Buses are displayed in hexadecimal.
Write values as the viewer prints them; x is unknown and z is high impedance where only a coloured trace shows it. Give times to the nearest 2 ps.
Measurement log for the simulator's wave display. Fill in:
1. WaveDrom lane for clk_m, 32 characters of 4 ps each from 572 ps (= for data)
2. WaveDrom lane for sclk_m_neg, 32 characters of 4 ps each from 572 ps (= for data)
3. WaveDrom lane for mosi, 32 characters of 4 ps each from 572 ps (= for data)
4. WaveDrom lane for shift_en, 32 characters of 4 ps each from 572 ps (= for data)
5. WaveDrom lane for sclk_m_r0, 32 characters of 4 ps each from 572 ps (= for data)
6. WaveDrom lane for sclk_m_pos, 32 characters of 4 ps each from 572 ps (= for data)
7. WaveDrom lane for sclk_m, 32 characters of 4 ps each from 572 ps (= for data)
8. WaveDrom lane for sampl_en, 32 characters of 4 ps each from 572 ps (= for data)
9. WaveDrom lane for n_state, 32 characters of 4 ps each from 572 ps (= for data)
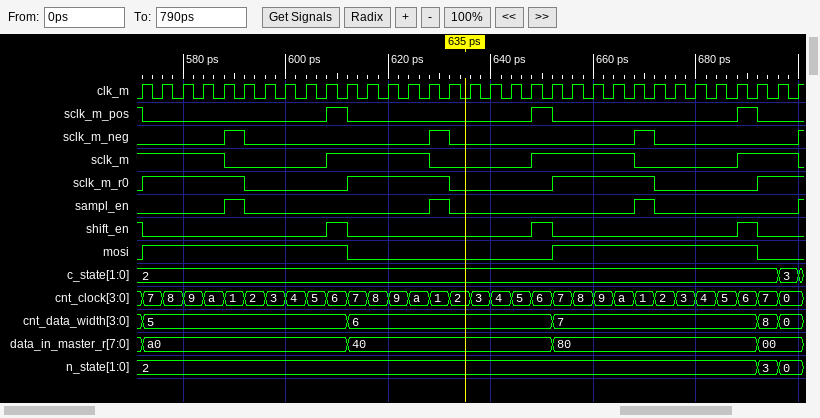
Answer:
{name: 'clk_m', wave: 'p...............................'}
{name: 'sclk_m_neg', wave: '0...10........10........10......'}
{name: 'mosi', wave: '1.........0.........1.........0.'}
{name: 'shift_en', wave: '0........10........10........10.'}
{name: 'sclk_m_r0', wave: '1....0....1....0....1....0....1.'}
{name: 'sclk_m_pos', wave: '0........10........10........10.'}
{name: 'sclk_m', wave: '1...0....1....0....1....0....1..'}
{name: 'sampl_en', wave: '0...10........10........10......'}
{name: 'n_state', wave: '=.............................==', data: '2 3 0'}
